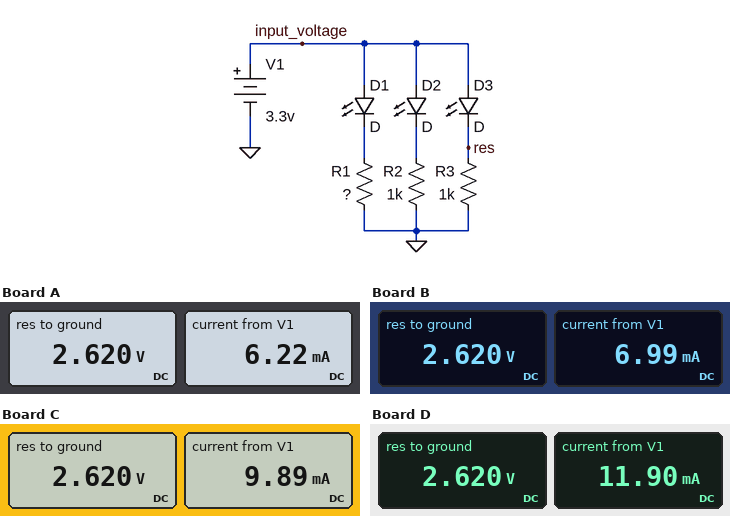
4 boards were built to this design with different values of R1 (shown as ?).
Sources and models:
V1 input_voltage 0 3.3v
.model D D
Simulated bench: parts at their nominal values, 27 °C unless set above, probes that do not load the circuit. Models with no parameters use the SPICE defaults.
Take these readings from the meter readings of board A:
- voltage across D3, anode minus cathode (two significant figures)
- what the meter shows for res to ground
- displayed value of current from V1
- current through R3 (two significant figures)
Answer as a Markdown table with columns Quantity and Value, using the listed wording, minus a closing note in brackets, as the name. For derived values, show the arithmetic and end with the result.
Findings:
| Quantity | Value |
|---|---|
| voltage across D3, anode minus cathode | 3.3 V - 2.62 V = 680 mV |
| what the meter shows for res to ground | 2.620 V |
| displayed value of current from V1 | 6.22 mA |
| current through R3 | (2.62 V) / 1 kΩ = 2.6 mA |
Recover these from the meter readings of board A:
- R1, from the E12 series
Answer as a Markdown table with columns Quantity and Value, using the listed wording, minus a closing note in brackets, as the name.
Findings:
| Quantity | Value |
|---|---|
| R1, from the E12 series | 2.7 kΩ |
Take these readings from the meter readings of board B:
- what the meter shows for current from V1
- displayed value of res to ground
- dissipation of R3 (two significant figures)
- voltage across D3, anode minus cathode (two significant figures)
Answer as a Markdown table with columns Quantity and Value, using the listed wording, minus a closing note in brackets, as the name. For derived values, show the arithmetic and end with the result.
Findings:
| Quantity | Value |
|---|---|
| what the meter shows for current from V1 | 6.99 mA |
| displayed value of res to ground | 2.620 V |
| dissipation of R3 | (2.62 V)^2 / 1 kΩ = 6.9 mW |
| voltage across D3, anode minus cathode | 3.3 V - 2.62 V = 680 mV |
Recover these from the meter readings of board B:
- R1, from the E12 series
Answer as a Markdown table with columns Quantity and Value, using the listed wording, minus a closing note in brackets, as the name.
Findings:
| Quantity | Value |
|---|---|
| R1, from the E12 series | 1.5 kΩ |
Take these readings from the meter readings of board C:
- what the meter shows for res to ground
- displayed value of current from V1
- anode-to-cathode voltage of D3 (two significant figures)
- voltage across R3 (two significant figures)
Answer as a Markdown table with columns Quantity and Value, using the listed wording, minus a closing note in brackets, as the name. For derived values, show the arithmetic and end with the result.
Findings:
| Quantity | Value |
|---|---|
| what the meter shows for res to ground | 2.620 V |
| displayed value of current from V1 | 9.89 mA |
| anode-to-cathode voltage of D3 | 3.3 V - 2.62 V = 680 mV |
| voltage across R3 | 2.62 V = 2.6 V |
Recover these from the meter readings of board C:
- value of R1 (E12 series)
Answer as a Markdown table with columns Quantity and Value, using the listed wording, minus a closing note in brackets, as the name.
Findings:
| Quantity | Value |
|---|---|
| value of R1 | 560 Ω |
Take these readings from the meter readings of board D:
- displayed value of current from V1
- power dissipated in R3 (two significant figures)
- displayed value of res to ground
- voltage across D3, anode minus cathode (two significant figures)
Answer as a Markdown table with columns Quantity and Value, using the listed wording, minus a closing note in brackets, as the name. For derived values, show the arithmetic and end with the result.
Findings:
| Quantity | Value |
|---|---|
| displayed value of current from V1 | 11.90 mA |
| power dissipated in R3 | (2.62 V)^2 / 1 kΩ = 6.9 mW |
| displayed value of res to ground | 2.620 V |
| voltage across D3, anode minus cathode | 3.3 V - 2.62 V = 680 mV |
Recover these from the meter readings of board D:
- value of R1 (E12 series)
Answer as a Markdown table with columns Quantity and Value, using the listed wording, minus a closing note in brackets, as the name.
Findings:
| Quantity | Value |
|---|---|
| value of R1 | 390 Ω |
